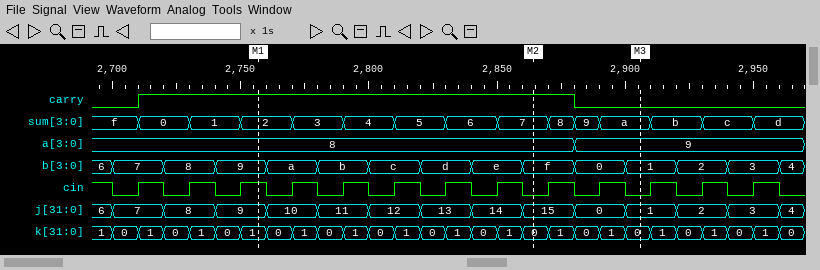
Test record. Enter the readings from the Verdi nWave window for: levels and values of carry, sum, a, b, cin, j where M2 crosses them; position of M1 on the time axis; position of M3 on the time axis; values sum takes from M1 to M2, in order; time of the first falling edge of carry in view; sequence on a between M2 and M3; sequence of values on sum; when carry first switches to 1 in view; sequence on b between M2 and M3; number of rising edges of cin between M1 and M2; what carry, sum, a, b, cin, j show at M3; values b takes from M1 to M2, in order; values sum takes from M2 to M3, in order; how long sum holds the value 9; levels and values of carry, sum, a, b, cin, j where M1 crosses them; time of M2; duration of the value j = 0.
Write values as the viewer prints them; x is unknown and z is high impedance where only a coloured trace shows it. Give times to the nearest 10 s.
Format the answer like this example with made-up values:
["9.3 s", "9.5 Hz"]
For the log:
["carry=1, sum=7, a=8, b=f, cin=0, j=15", "2760 s", "2910 s", "2, 3, 4, 5, 6, 7", "2880 s", "8, 9", "f, 0, 1, 2, 3, 4, 5, 6, 7, 8, 9, a, b, c, d", "2710 s", "f, 0, 1", "5", "carry=0, sum=a, a=9, b=1, cin=0, j=1", "9, a, b, c, d, e, f", "7, 8, 9, a", "10 s", "carry=1, sum=2, a=8, b=9, cin=1, j=9", "2860 s", "20 s"]
